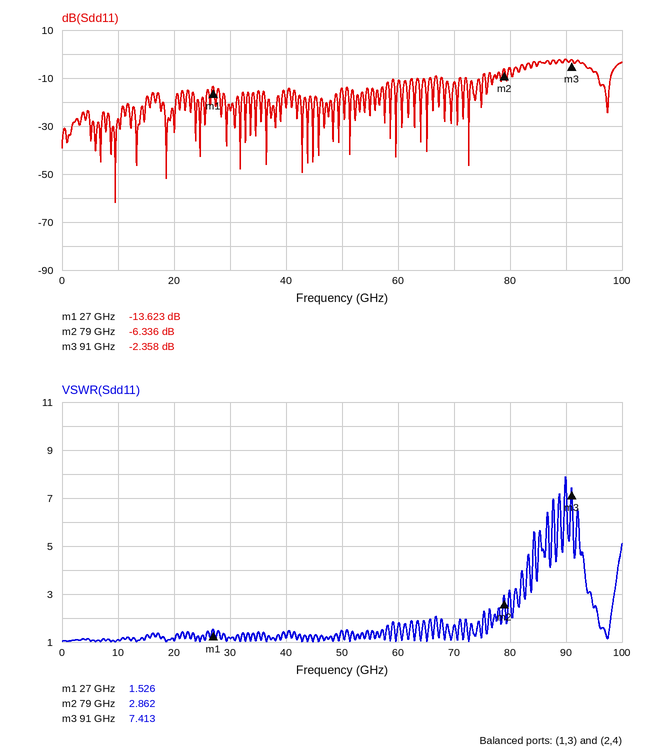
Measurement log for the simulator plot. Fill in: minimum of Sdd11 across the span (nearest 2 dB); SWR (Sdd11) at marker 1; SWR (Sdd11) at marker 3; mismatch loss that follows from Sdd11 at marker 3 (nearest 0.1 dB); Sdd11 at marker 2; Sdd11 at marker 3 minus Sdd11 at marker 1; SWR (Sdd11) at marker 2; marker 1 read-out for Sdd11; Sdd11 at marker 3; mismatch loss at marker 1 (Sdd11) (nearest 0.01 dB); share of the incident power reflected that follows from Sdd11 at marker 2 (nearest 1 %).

-62 dB
1.526
7.413
3.8 dB
-6.336 dB
11.265 dB
2.862
-13.623 dB
-2.358 dB
0.19 dB
23 %
